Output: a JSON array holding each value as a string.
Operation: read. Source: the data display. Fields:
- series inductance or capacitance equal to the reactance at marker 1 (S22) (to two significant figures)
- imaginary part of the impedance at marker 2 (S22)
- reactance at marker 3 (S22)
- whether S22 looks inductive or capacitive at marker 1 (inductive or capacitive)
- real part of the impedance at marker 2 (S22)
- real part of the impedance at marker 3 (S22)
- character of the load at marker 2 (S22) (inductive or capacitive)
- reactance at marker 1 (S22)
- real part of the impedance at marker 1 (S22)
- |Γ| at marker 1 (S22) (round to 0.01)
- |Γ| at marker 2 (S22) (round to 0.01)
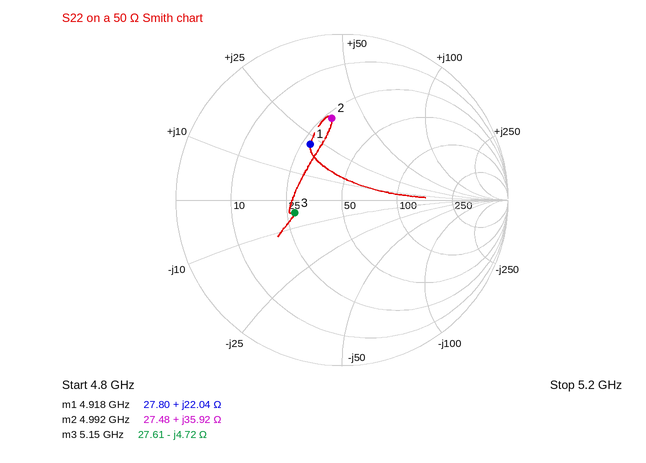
["710 pH", "+35.92 Ω", "-4.72 Ω", "inductive", "27.48 Ω", "27.61 Ω", "inductive", "+22.04 Ω", "27.80 Ω", "0.39", "0.50"]
